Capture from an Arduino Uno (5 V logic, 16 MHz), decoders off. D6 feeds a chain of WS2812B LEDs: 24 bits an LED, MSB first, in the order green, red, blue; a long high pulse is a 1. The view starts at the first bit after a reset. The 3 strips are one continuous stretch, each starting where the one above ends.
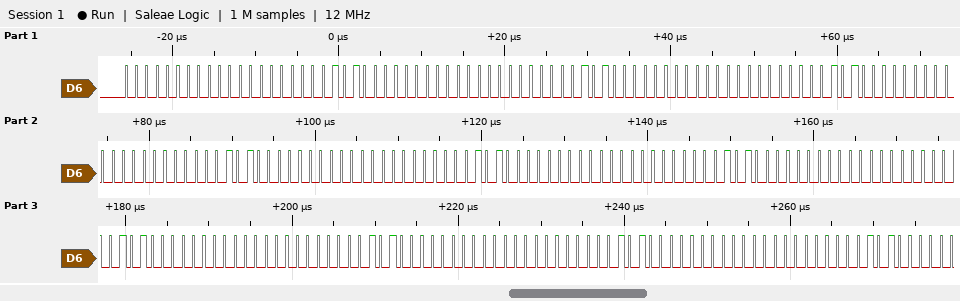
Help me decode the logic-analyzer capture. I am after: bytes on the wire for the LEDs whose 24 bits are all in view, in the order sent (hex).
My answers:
00 00 0A 00 00 0A 00 00 0A 00 00 0A 00 00 0A 00 00 0A 00 00 0A 00 00 0A 00 00 0A 00 00 0A
